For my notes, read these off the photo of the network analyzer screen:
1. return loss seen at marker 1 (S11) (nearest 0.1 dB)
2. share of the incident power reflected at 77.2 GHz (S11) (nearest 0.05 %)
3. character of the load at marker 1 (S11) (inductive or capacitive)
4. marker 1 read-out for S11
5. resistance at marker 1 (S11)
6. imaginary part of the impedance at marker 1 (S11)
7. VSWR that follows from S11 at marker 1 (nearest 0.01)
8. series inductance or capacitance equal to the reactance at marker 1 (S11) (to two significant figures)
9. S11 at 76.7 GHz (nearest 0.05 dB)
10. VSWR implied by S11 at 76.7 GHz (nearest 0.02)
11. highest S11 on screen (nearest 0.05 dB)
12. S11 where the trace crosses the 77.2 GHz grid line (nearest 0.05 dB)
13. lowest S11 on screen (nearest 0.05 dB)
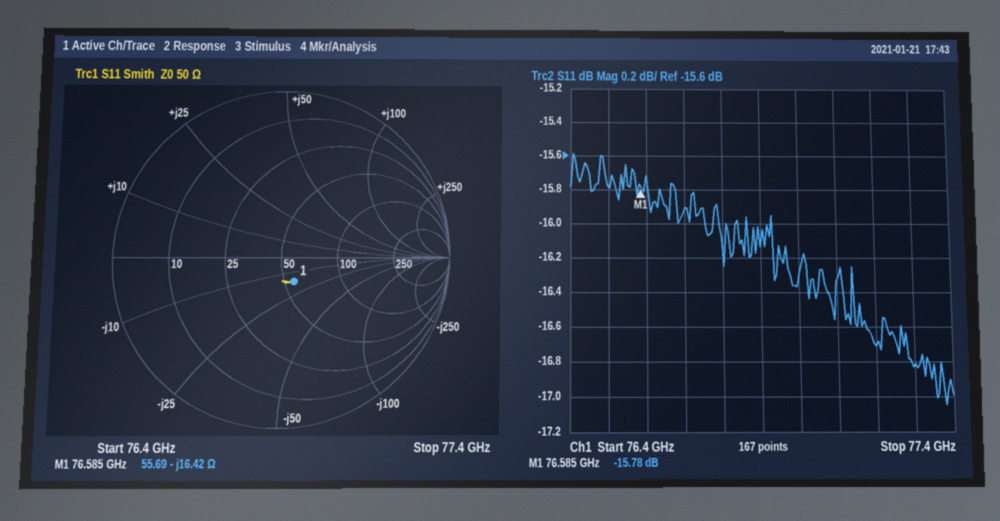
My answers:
15.8 dB
2.15 %
capacitive
-15.78 dB
55.69 Ω
-16.42 Ω
1.39
130 fF
-15.90 dB
1.38
-15.60 dB
-16.70 dB
-17.05 dB
